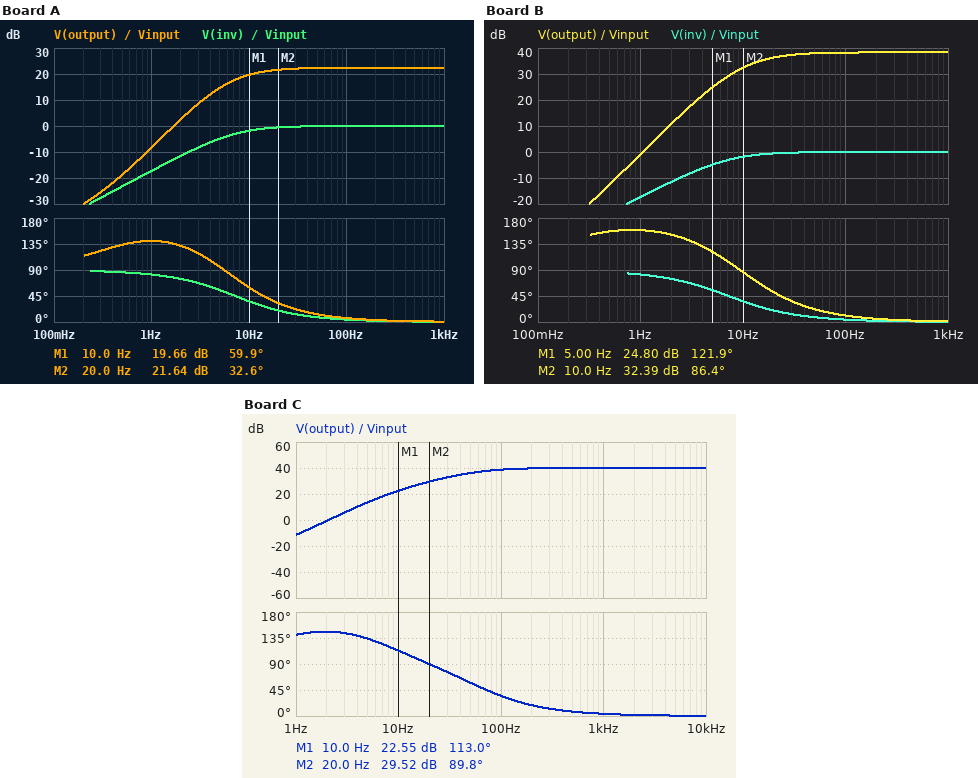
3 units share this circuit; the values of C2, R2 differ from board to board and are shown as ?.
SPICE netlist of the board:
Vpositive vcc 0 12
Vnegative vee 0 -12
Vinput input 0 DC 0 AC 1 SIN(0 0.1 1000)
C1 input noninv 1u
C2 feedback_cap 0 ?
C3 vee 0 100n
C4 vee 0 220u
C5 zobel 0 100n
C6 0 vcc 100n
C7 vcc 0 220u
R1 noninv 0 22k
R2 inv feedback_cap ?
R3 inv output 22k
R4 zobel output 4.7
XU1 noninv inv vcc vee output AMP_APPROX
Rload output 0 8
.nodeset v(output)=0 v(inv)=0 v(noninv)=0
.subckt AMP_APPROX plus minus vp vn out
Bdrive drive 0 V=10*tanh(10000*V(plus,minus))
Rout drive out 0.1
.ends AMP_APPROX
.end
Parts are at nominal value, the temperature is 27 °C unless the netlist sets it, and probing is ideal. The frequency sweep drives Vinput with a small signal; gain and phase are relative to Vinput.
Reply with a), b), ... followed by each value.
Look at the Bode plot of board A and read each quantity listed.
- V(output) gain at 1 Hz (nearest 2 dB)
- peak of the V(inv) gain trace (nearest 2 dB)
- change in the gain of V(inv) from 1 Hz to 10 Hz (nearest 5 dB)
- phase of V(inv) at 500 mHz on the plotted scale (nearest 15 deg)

a) -8 dB
b) 0 dB
c) 15 dB
d) 90 deg
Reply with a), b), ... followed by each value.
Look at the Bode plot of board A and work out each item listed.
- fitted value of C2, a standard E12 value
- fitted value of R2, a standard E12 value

a) 18 µF
b) 1.8 kΩ
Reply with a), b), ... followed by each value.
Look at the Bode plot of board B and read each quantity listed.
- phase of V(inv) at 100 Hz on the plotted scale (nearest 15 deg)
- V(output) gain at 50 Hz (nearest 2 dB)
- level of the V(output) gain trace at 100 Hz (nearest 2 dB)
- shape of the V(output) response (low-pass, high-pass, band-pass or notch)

a) 0 deg
b) 38 dB
c) 38 dB
d) high-pass
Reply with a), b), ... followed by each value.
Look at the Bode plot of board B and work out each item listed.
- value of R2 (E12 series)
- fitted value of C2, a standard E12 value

a) 270 Ω
b) 47 µF
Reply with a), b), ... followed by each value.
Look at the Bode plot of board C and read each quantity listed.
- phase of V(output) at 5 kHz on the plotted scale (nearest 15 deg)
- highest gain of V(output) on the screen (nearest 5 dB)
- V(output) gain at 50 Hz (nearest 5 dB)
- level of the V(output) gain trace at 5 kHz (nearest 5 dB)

a) 0 deg
b) 40 dB
c) 35 dB
d) 40 dB
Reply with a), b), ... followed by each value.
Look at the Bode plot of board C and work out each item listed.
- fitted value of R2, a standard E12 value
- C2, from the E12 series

a) 220 Ω
b) 12 µF
